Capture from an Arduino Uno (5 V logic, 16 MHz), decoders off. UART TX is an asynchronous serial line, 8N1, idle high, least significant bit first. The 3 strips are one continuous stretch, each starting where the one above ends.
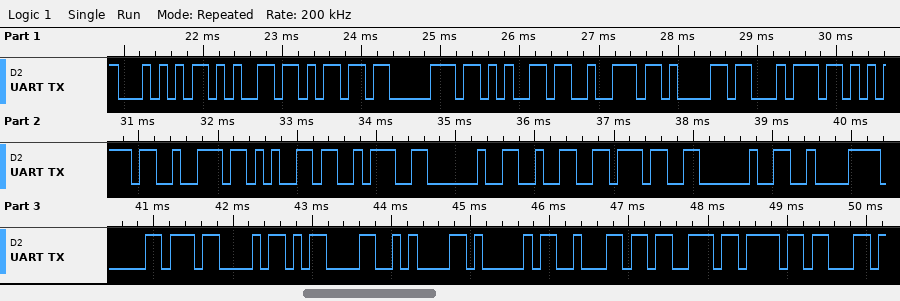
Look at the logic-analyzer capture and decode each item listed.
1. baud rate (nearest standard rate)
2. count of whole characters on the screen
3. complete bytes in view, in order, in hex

9600 baud
25
54 65 6D 70 65 72 61 74 75 72 65 3A 20 32 37 20 C2 B0 43 0D 0A 41 62 73 6F
